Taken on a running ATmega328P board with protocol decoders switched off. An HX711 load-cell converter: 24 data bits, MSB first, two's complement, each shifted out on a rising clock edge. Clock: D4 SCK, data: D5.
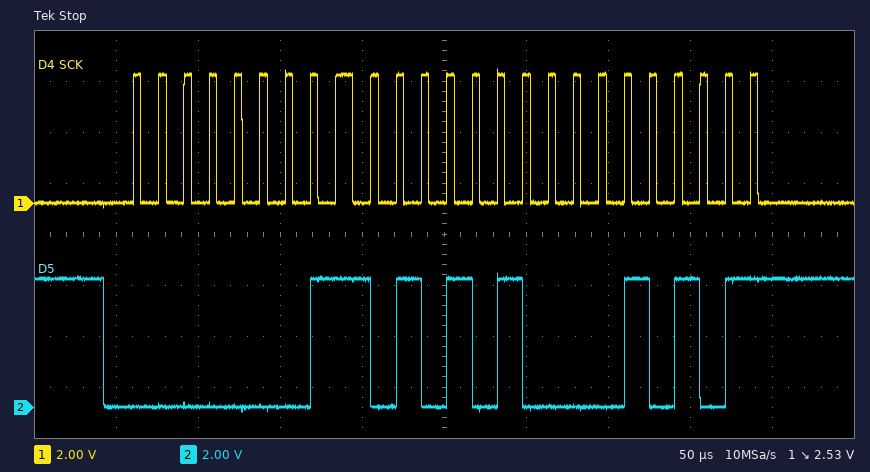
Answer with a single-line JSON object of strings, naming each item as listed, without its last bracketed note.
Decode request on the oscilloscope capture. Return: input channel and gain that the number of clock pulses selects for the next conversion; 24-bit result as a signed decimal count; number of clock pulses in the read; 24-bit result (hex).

{"input channel and gain that the number of clock pulses selects for the next conversion": "channel A, gain 128", "24-bit result as a signed decimal count": "109077", "number of clock pulses in the read": "25", "24-bit result": "0x01AA15"}
